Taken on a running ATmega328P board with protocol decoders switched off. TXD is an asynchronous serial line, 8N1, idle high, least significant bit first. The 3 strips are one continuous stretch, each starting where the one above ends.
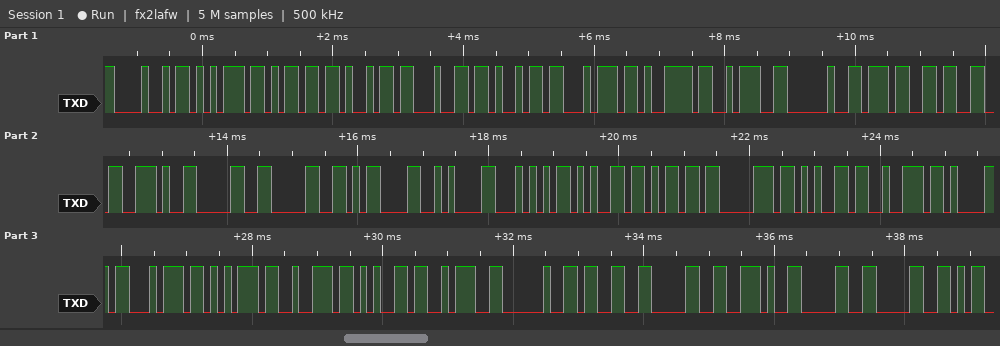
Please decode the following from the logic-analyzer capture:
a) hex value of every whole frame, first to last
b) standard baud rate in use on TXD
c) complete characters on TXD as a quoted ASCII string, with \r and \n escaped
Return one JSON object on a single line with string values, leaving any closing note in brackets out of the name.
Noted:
{"hex value of every whole frame, first to last": "48 75 6D 69 64 69 74 79 3A 20 37 33 2E 30 30 0D 0A 54 65 6D 70 65 72 61 74 75 72 65 3A 20 33 30 2E 30 30", "standard baud rate in use on TXD": "9600 baud", "complete characters on TXD as a quoted ASCII string, with \\r and \\n escaped": "\"Humidity: 73.00\\r\\nTemperature: 30.00\""}
